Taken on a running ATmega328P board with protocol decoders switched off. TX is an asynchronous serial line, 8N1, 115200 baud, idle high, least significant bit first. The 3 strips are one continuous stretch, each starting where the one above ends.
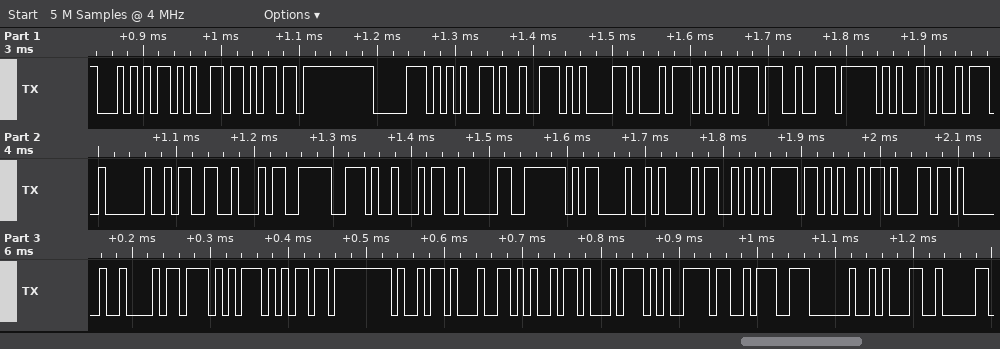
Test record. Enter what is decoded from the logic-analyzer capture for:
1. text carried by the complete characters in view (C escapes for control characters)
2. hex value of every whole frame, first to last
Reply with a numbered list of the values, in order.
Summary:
1. "Temperature: 34.40\r\nSoil humidity: 1"
2. 54 65 6D 70 65 72 61 74 75 72 65 3A 20 33 34 2E 34 30 0D 0A 53 6F 69 6C 20 68 75 6D 69 64 69 74 79 3A 20 31
